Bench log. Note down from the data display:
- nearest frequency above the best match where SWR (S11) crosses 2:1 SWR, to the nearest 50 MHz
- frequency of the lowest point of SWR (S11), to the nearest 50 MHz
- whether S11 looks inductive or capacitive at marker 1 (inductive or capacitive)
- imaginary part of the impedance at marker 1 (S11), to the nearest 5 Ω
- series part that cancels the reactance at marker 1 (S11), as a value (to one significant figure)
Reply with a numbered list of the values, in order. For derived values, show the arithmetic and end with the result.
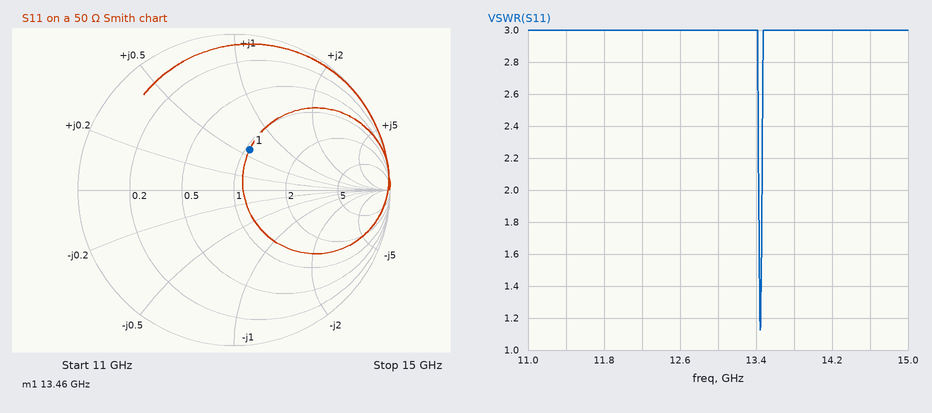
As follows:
1. 13.45 GHz
2. 13.45 GHz
3. inductive
4. +30 Ω
5. C = 1/(2π × 13.46 GHz × 30 Ω) ≈ 394 fF, so 400 fF to one significant figure
